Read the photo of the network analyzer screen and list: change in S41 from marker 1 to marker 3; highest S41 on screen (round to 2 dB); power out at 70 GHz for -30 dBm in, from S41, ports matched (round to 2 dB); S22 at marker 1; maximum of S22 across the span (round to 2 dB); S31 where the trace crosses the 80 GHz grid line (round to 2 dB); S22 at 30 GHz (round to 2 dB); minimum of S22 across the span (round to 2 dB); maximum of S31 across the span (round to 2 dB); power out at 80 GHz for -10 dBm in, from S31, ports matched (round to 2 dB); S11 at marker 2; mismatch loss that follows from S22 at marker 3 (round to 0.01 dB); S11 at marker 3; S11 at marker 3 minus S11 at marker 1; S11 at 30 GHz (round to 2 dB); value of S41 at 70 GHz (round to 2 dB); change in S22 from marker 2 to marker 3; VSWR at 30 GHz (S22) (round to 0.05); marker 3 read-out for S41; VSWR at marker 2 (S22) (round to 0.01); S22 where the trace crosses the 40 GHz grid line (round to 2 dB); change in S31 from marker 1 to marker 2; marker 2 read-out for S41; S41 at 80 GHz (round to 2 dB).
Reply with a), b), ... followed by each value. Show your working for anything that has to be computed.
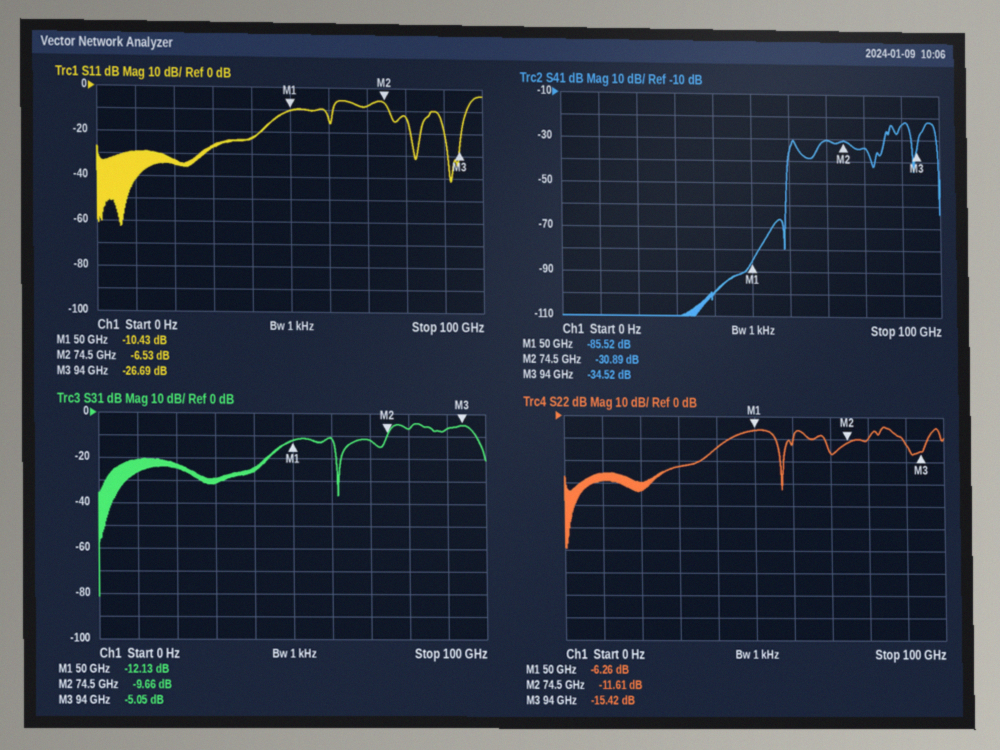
a) -34.52 − (-85.52) = 51.00 dB
b) -22 dB
c) -30 dBm + (-30 dB) = -60 dBm
d) -6.26 dB
e) -4 dB
f) -6 dB
g) -22 dB
h) -60 dB
i) -4 dB
j) -10 dBm + (-6 dB) = -16 dBm
k) -6.53 dB
l) −10 log10(1 − 10^(-15.42/10)) ≈ 0.13 dB
m) -26.69 dB
n) -26.69 − (-10.43) = -16.26 dB
o) -26 dB
p) -30 dB
q) -15.42 − (-11.61) = -3.81 dB
r) |Γ| = 10^(-22/20) = 0.0794; VSWR = (1 + 0.0794)/(1 − 0.0794) ≈ 1.17, so 1.15 to the nearest 0.05
s) -34.52 dB
t) (1 + 0.2627)/(1 − 0.2627) ≈ 1.71
u) -14 dB
v) -9.66 − (-12.13) = 2.47 dB
w) -30.89 dB
x) -34 dB
